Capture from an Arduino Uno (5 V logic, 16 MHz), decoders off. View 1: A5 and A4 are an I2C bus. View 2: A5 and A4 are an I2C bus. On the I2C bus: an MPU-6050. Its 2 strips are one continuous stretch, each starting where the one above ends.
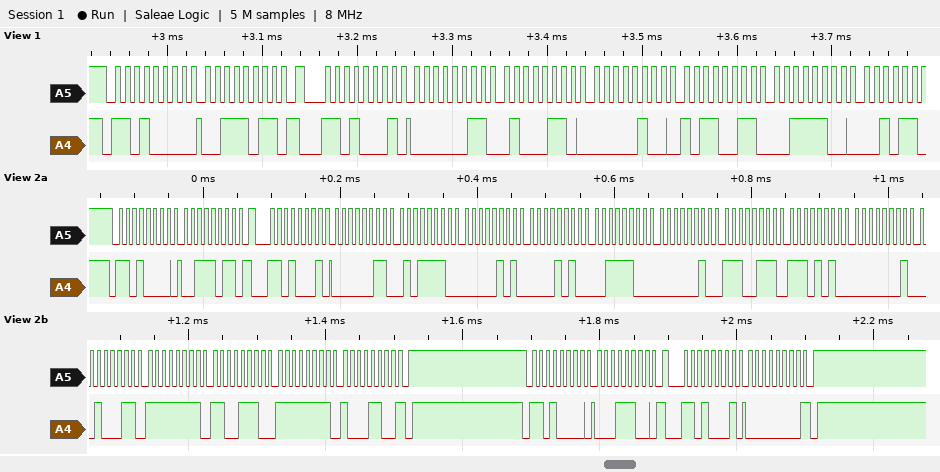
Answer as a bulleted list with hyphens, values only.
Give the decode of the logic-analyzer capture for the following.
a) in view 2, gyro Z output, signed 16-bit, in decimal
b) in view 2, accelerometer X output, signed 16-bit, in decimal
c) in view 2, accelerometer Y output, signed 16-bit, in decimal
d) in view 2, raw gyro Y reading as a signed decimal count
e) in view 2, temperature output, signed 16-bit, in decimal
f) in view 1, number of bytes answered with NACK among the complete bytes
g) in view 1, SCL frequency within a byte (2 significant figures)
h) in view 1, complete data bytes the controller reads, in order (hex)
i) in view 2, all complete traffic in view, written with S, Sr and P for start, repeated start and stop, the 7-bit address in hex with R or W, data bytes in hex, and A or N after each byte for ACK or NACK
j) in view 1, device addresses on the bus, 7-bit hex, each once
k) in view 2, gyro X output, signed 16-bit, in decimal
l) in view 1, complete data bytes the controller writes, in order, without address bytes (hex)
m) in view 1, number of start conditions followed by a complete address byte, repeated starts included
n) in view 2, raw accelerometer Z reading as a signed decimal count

- -116
- 862
- 1290
- -50
- -6166
- 0
- 100 kHz
- 03 46 04 B3 3C
- S 68W A 3B A Sr 68R A 03 A 5E A 05 A 0A A 3C A 02 A E7 A EA A 01 A 23 A FF A CE A FF A 8C N P S 68W A 1C A Sr 68R A 00 N P
- 0x68
- 291
- 3B
- 2
- 15362
